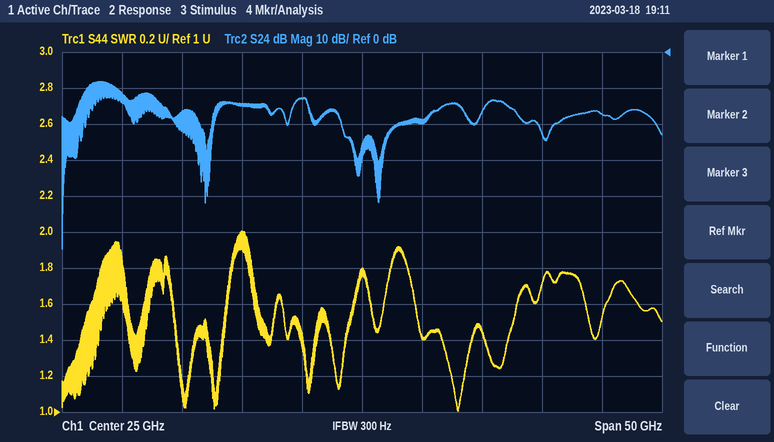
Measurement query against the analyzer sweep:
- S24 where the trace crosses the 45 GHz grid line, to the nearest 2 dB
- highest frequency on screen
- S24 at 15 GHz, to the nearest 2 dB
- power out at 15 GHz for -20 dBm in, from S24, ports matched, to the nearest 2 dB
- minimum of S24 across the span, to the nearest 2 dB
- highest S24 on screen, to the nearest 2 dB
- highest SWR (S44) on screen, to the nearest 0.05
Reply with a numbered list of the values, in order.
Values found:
1. -18 dB
2. 50 GHz
3. -14 dB
4. -34 dBm
5. -54 dB
6. -8 dB
7. 2.00
